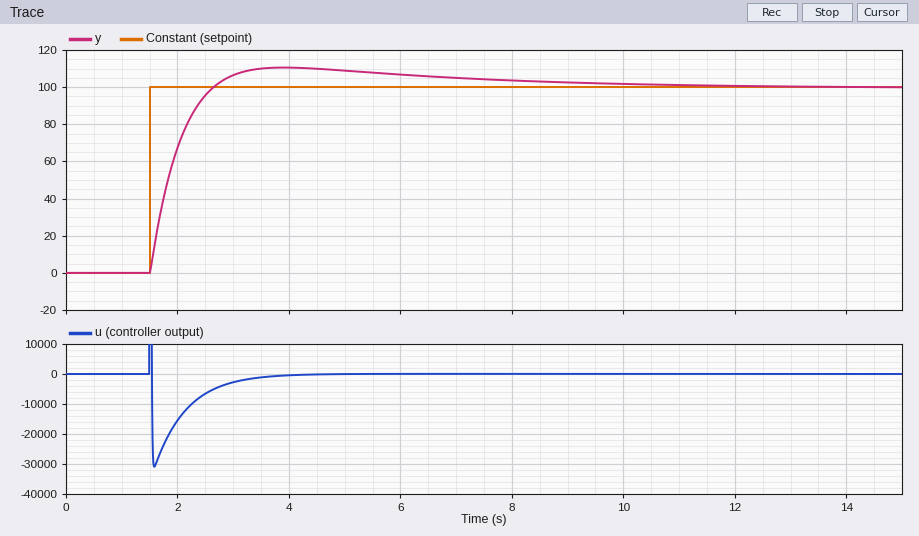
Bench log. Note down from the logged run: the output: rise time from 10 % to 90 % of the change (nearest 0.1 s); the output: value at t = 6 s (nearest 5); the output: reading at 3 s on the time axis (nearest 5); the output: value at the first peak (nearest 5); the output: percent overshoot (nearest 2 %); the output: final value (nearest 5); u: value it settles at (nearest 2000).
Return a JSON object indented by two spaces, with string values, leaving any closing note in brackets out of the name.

{
  "the output: rise time from 10 % to 90 % of the change": "0.8 s",
  "the output: value at t = 6 s": "105",
  "the output: reading at 3 s on the time axis": "105",
  "the output: value at the first peak": "110",
  "the output: percent overshoot": "10 %",
  "the output: final value": "100",
  "u: value it settles at": "0"
}
